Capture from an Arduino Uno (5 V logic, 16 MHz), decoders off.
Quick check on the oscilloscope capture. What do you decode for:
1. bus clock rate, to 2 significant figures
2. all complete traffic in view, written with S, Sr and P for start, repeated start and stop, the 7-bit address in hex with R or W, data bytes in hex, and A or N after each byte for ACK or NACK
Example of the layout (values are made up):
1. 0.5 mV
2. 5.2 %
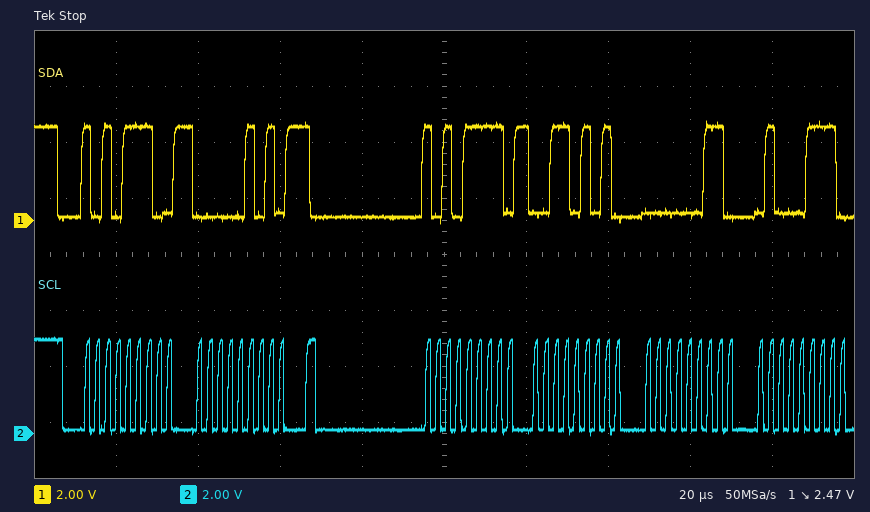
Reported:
1. 400 kHz
2. S 57W A 05 A Sr 57R A 35 A 03 A 47 A
